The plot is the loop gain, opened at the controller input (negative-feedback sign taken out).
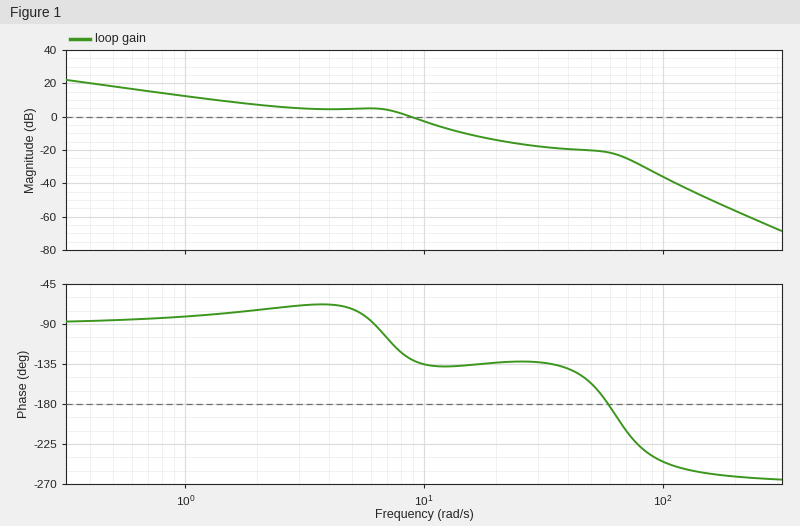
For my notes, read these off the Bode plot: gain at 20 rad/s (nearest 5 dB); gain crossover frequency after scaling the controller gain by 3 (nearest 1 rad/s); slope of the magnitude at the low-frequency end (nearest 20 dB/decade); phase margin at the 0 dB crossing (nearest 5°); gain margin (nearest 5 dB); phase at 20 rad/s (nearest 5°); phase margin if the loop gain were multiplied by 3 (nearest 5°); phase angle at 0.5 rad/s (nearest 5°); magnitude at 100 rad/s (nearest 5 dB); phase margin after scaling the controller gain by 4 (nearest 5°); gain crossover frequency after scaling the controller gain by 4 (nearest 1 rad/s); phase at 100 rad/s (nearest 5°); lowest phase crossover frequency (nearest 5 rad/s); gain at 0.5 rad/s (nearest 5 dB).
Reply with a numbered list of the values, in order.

1. -15 dB
2. 14 rad/s
3. -20 dB/decade
4. 50°
5. 20 dB
6. -135°
7. 45°
8. -85°
9. -35 dB
10. 45°
11. 17 rad/s
12. -245°
13. 60 rad/s
14. 20 dB
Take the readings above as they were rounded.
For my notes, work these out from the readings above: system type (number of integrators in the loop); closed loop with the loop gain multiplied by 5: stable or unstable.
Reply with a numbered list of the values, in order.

1. 1
2. stable
